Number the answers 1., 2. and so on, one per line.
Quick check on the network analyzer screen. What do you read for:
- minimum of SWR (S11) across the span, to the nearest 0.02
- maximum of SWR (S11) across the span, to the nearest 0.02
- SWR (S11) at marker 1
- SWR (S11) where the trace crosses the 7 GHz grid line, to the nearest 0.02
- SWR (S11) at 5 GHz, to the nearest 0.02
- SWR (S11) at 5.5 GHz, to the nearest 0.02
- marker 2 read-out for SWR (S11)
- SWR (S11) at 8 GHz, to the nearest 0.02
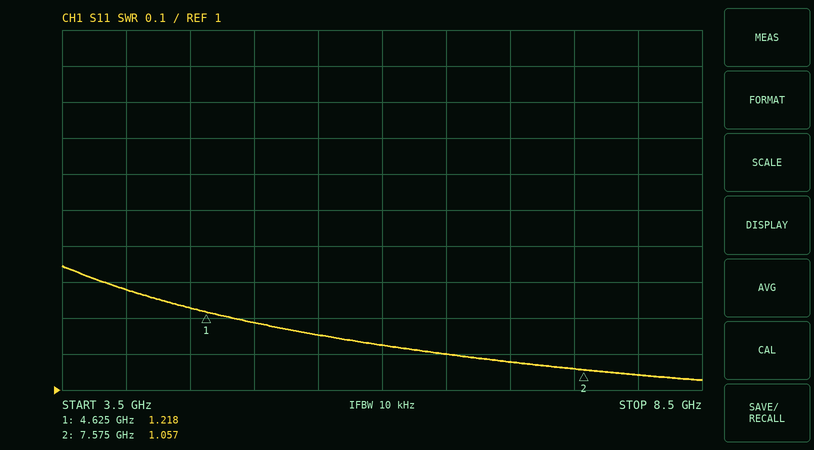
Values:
1. 1.02
2. 1.34
3. 1.218
4. 1.08
5. 1.18
6. 1.16
7. 1.057
8. 1.04
